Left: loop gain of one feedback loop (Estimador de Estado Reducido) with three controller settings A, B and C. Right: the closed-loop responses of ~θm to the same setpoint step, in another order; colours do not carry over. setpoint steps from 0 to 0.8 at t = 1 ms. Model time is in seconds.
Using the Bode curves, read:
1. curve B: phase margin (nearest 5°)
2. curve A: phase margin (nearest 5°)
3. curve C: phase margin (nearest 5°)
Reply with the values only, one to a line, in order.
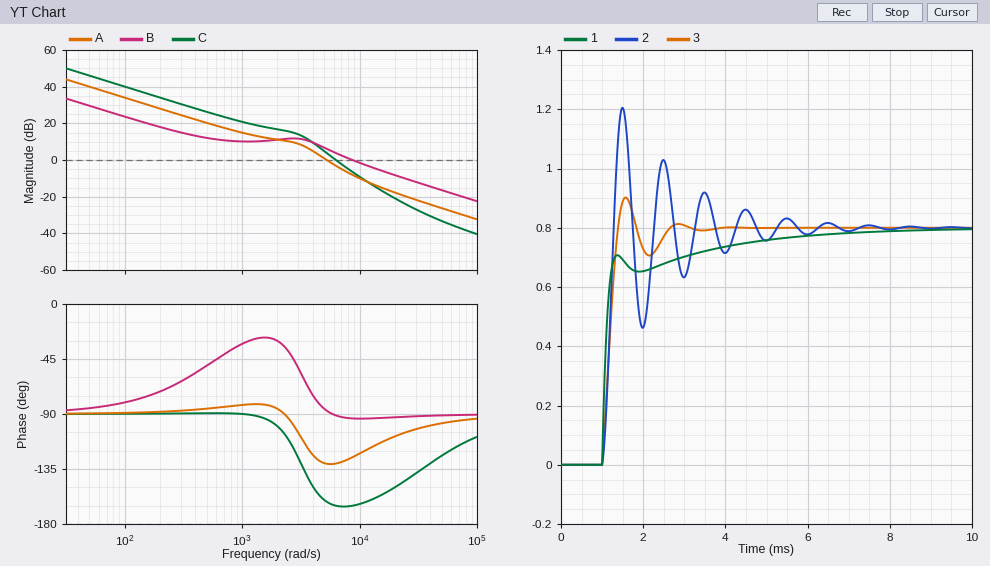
85°
50°
15°
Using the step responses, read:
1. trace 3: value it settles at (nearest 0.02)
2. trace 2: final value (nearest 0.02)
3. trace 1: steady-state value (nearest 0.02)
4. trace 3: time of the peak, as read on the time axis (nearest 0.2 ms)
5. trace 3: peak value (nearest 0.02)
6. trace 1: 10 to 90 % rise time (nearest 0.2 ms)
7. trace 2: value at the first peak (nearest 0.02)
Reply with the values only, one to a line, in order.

0.80
0.80
0.80
1.6 ms
0.90
2.4 ms
1.20
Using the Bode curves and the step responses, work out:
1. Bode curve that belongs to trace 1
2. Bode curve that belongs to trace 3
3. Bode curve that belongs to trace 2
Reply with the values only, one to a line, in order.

B
A
C
